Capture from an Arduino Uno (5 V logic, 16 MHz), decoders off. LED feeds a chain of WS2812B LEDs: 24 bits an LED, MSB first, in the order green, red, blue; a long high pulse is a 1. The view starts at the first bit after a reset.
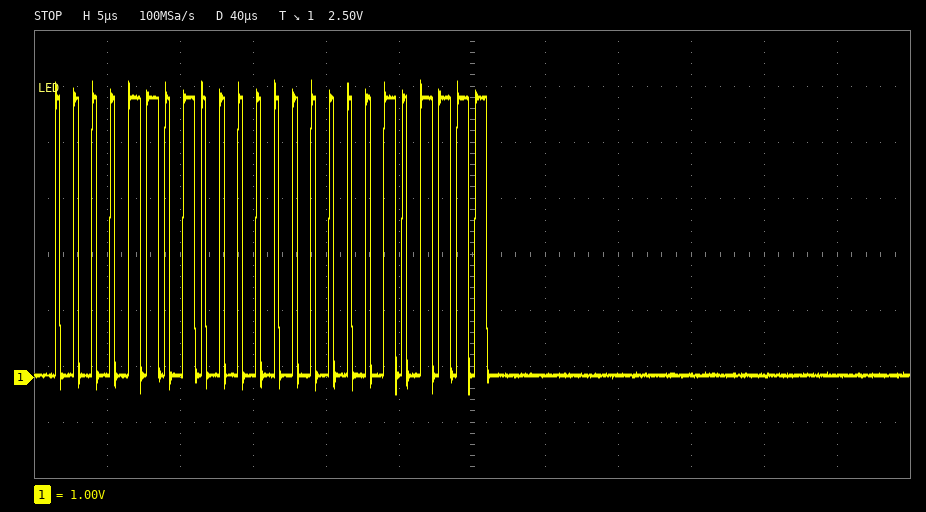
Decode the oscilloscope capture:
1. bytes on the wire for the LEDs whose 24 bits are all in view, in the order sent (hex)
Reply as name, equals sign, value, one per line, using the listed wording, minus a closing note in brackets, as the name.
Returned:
bytes on the wire for the LEDs whose 24 bits are all in view, in the order sent = 0D 00 2F
